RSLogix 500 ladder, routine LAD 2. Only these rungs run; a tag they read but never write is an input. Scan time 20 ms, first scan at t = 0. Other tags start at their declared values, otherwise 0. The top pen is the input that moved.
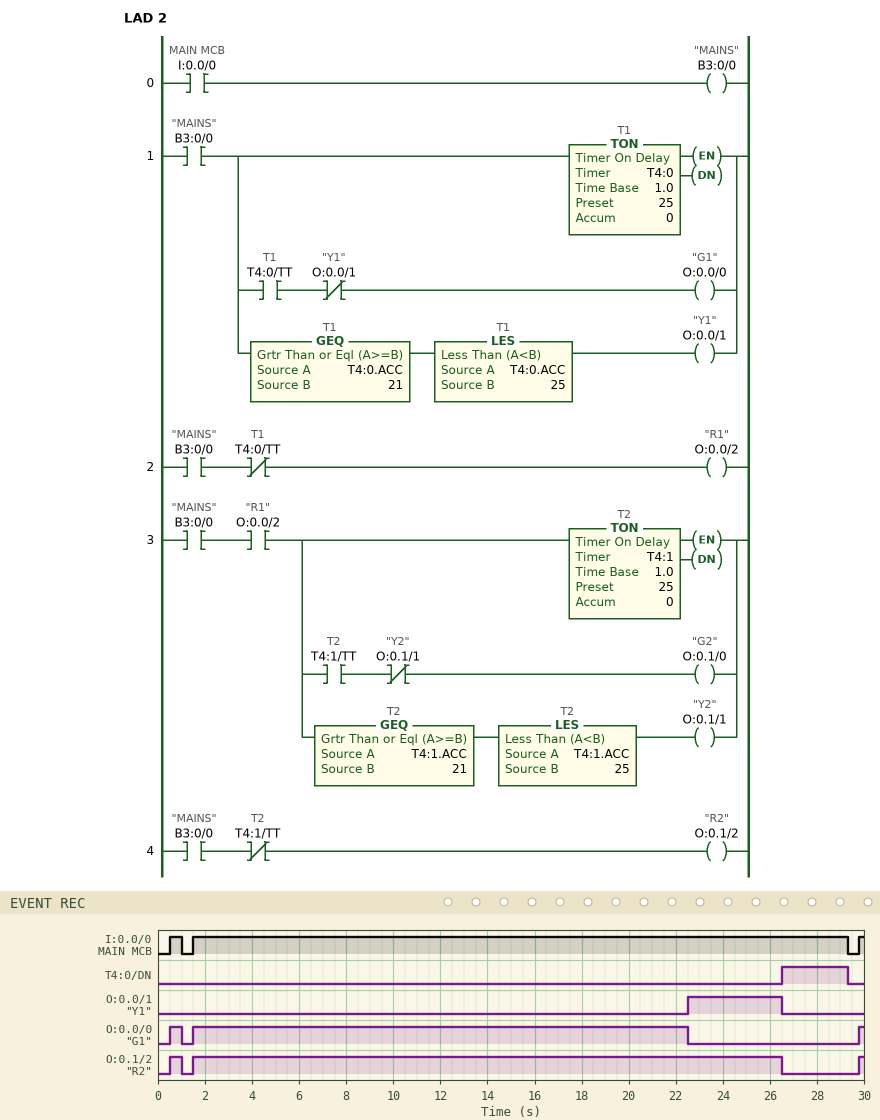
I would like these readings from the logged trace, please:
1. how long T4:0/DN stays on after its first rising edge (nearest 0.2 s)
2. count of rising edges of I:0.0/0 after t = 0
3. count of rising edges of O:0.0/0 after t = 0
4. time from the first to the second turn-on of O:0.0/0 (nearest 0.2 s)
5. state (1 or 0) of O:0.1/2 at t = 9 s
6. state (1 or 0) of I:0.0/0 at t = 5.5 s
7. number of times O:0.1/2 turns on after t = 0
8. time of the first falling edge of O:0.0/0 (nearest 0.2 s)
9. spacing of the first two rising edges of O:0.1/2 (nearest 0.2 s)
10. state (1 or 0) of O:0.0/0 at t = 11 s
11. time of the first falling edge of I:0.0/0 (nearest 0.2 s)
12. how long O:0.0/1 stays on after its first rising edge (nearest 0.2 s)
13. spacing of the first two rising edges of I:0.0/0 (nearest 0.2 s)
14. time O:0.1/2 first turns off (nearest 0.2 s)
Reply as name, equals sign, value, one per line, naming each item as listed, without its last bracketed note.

how long T4:0/DN stays on after its first rising edge = 2.8 s
count of rising edges of I:0.0/0 after t = 0 = 3
count of rising edges of O:0.0/0 after t = 0 = 3
time from the first to the second turn-on of O:0.0/0 = 1.0 s
state (1 or 0) of O:0.1/2 at t = 9 s = 1
state (1 or 0) of I:0.0/0 at t = 5.5 s = 1
number of times O:0.1/2 turns on after t = 0 = 3
time of the first falling edge of O:0.0/0 = 1.0 s
spacing of the first two rising edges of O:0.1/2 = 1.0 s
state (1 or 0) of O:0.0/0 at t = 11 s = 1
time of the first falling edge of I:0.0/0 = 1.0 s
how long O:0.0/1 stays on after its first rising edge = 4.0 s
spacing of the first two rising edges of I:0.0/0 = 1.0 s
time O:0.1/2 first turns off = 1.0 s
